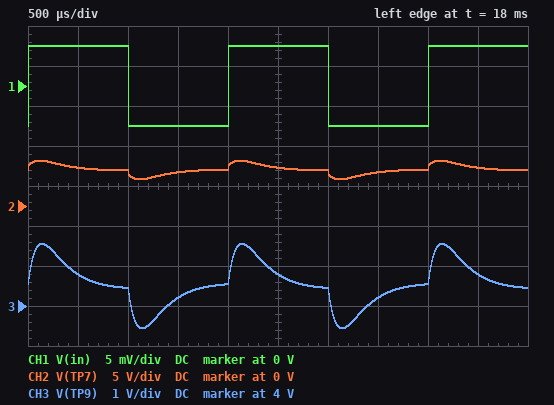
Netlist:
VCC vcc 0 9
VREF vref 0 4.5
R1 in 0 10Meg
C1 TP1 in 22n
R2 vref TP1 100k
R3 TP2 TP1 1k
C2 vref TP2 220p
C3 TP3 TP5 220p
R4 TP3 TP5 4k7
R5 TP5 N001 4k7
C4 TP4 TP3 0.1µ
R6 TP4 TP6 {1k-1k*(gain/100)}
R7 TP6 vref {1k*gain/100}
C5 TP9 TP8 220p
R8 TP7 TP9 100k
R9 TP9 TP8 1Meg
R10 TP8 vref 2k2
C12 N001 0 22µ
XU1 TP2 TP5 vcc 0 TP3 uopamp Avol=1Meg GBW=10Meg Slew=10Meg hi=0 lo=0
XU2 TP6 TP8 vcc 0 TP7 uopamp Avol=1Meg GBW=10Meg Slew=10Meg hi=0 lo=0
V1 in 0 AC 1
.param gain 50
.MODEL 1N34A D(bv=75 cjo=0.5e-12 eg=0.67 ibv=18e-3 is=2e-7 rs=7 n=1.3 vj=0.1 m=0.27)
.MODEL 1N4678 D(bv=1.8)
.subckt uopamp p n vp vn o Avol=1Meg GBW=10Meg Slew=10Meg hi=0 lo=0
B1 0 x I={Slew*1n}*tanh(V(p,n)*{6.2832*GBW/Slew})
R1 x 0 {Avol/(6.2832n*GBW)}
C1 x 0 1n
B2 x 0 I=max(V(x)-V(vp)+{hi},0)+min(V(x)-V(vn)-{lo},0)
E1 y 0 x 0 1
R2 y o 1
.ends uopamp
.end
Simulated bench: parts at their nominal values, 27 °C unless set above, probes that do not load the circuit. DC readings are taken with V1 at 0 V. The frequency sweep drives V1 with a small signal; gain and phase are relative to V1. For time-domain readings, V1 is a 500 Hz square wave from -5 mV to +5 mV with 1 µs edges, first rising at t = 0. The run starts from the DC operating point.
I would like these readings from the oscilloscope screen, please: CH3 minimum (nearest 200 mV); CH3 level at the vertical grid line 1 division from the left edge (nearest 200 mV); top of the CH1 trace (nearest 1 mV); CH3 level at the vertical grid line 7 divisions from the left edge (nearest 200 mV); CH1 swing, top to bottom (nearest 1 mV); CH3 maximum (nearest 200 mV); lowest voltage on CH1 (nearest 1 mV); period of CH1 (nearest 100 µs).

3.4 V
4.8 V
5 mV
4.2 V
10 mV
5.6 V
-5 mV
2.0 ms
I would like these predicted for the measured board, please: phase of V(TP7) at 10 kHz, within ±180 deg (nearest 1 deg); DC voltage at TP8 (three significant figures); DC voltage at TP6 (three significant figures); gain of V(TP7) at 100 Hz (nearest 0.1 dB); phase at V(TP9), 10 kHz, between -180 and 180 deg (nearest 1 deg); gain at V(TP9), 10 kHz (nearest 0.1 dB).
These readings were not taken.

-30 deg
4.50 V
4.50 V
28.0 dB
-80 deg
29.8 dB
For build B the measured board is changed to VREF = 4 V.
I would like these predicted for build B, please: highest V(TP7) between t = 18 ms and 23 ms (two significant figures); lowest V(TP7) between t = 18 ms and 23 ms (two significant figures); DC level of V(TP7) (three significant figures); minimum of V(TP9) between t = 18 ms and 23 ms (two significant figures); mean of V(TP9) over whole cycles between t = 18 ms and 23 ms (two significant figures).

5.2 V
2.8 V
4.00 V
2.9 V
4.0 V
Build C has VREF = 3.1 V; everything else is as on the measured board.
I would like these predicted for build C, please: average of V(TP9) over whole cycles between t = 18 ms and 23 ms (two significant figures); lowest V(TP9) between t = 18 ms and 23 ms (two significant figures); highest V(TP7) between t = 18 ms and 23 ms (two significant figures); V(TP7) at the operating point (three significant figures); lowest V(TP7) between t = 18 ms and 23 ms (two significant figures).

3.1 V
2.0 V
4.3 V
3.10 V
1.9 V
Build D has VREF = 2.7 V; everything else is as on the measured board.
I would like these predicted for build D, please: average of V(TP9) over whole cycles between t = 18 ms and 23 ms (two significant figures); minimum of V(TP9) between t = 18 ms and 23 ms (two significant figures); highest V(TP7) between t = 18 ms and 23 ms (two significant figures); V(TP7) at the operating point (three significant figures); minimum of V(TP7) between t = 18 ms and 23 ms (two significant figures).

2.7 V
1.6 V
3.9 V
2.70 V
1.5 V
